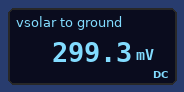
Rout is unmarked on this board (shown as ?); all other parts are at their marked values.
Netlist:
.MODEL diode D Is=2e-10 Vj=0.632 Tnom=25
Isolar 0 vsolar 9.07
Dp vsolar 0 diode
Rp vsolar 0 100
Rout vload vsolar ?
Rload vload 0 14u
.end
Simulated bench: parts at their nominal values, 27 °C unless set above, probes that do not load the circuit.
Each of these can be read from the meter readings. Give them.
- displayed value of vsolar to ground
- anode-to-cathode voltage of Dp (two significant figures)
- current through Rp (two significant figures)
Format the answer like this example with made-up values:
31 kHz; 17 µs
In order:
299.3 mV; 300 mV; 3.0 mA
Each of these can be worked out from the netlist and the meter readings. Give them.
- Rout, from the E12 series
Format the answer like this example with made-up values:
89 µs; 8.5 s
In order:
0.033 Ω
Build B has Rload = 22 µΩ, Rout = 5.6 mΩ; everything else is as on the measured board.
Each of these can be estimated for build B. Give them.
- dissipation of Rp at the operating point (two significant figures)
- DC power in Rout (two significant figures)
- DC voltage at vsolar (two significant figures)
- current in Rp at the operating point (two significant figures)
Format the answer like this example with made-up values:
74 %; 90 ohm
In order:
26 µW; 460 mW; 51 mV; 510 µA
